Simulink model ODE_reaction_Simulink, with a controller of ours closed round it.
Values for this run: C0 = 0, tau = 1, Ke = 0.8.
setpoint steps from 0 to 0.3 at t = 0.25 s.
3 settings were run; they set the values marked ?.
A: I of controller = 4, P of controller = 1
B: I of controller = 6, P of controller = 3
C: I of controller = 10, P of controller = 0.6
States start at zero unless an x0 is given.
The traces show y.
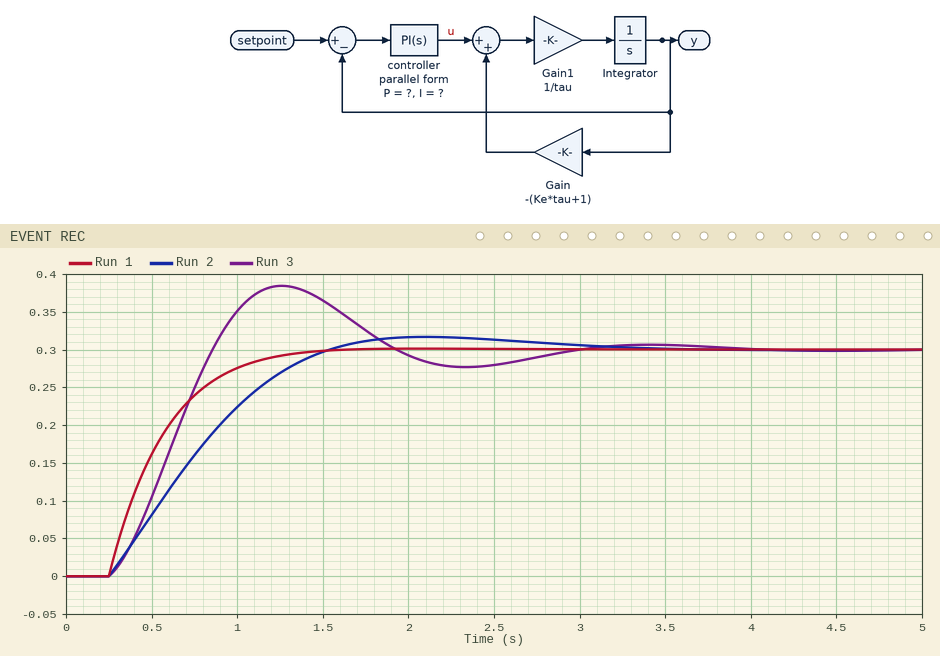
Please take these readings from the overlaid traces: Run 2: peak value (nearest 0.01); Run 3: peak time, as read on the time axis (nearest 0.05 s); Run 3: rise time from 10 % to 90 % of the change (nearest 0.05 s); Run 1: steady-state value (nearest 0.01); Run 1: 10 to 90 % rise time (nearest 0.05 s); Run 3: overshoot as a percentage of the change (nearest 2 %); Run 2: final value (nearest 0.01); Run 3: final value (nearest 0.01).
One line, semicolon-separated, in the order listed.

0.32; 1.25 s; 0.45 s; 0.30; 0.65 s; 28 %; 0.30; 0.30
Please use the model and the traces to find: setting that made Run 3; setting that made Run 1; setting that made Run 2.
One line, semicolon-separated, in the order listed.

C; B; A
